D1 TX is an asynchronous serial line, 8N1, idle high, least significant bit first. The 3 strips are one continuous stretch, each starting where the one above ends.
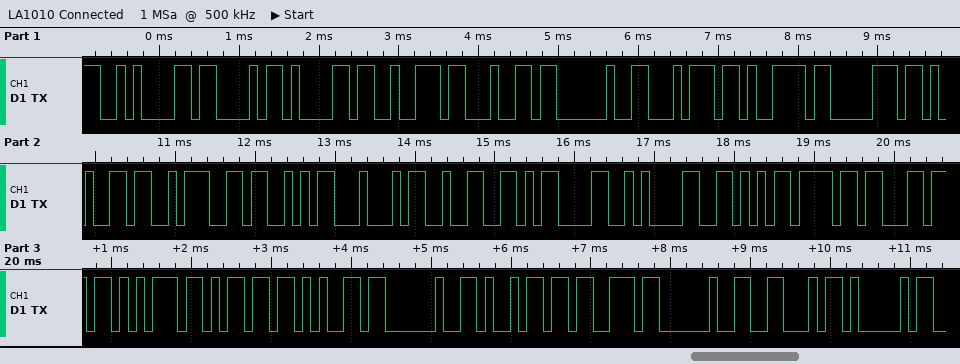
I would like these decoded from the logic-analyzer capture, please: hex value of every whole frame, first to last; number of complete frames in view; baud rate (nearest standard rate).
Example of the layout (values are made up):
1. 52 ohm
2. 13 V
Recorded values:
1. 0A 43 61 72 64 20 74 79 70 65 3A 53 44 32 0D 0A 56 6F 6C 75 6D 65 20 69 73 20 46 41
2. 28
3. 9600 baud
